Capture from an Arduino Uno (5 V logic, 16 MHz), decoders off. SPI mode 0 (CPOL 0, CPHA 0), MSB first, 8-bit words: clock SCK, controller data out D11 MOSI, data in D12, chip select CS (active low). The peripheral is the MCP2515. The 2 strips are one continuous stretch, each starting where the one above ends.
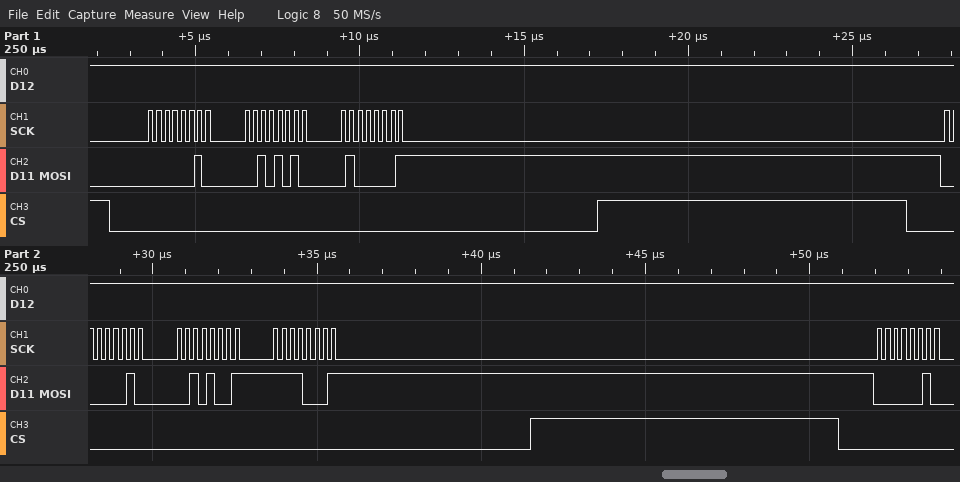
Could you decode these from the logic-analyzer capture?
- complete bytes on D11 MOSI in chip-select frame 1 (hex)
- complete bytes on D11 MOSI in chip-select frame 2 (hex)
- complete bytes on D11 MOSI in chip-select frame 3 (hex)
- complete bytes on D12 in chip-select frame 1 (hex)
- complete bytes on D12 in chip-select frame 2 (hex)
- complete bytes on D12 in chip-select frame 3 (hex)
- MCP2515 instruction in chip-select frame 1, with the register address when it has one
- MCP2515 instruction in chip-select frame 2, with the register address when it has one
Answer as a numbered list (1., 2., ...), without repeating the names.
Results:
1. 02 2A 41
2. 02 29 F1
3. 02
4. FF FF FF
5. FF FF FF
6. FF
7. WRITE 0x2A
8. WRITE 0x29
